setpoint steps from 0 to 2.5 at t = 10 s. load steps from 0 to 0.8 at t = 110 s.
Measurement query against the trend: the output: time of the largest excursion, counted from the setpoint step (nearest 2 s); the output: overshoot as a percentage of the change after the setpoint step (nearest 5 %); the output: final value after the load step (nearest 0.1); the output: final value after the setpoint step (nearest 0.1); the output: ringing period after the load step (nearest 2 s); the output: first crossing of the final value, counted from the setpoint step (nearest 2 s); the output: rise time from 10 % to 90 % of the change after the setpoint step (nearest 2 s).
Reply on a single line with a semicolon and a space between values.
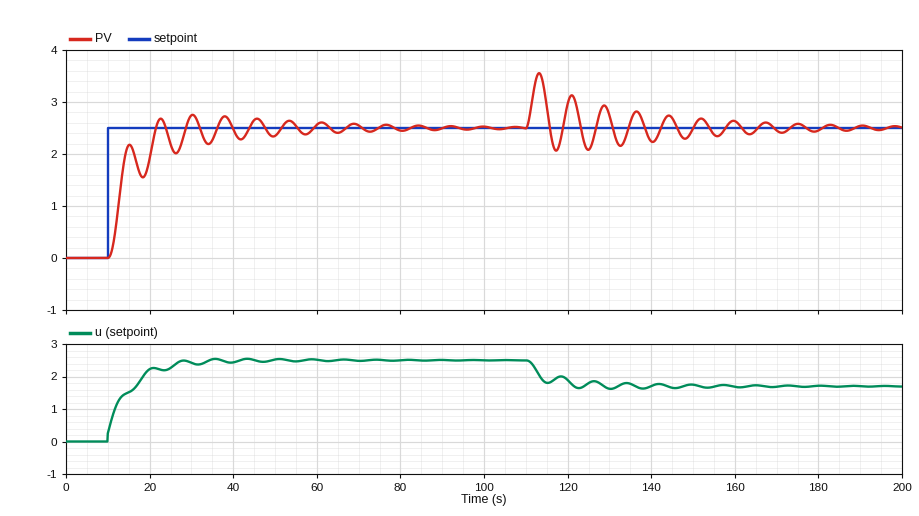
20 s; 10 %; 2.5; 2.5; 8 s; 12 s; 10 s
